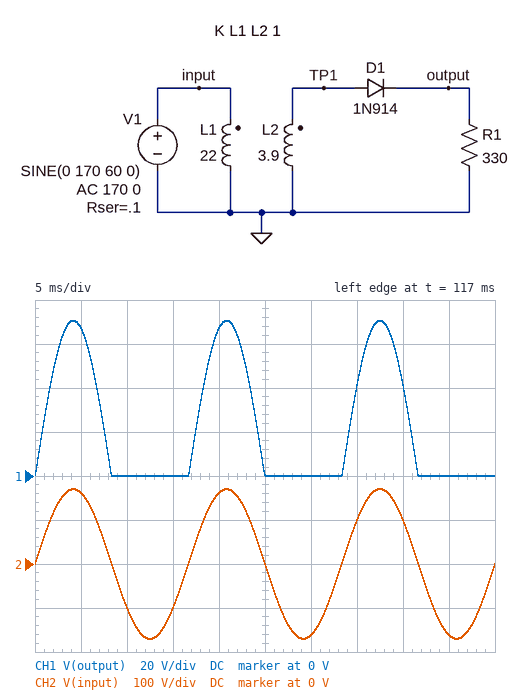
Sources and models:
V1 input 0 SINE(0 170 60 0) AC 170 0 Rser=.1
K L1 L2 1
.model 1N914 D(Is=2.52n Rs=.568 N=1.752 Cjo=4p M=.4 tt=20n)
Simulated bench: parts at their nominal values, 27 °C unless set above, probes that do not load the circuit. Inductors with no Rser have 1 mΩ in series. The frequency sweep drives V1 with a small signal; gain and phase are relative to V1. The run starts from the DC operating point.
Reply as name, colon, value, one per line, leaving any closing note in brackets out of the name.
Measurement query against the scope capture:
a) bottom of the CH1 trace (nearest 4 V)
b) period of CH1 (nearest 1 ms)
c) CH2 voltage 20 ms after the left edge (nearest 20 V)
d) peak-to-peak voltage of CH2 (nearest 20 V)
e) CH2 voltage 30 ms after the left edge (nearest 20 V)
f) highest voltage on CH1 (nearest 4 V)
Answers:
bottom of the CH1 trace: 0 V
period of CH1: 17 ms
CH2 voltage 20 ms after the left edge: 160 V
peak-to-peak voltage of CH2: 340 V
CH2 voltage 30 ms after the left edge: -160 V
highest voltage on CH1: 72 V
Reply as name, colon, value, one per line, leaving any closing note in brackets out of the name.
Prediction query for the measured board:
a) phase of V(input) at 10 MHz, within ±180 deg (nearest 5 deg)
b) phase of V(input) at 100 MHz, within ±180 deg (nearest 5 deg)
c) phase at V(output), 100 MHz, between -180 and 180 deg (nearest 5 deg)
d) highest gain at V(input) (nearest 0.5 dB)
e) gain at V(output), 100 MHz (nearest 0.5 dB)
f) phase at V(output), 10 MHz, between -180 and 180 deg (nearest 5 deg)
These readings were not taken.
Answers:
phase of V(input) at 10 MHz, within ±180 deg: 0 deg
phase of V(input) at 100 MHz, within ±180 deg: 0 deg
phase at V(output), 100 MHz, between -180 and 180 deg: 50 deg
highest gain at V(input): 0 dB
gain at V(output), 100 MHz: -11.5 dB
phase at V(output), 10 MHz, between -180 and 180 deg: 85 deg
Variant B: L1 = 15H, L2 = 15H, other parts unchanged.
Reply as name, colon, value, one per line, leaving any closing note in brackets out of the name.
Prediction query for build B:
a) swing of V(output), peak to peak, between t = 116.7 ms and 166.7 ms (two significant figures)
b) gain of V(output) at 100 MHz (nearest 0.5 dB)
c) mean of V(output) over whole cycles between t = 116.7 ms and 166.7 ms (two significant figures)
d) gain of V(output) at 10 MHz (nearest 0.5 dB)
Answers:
swing of V(output), peak to peak, between t = 116.7 ms and 166.7 ms: 170 V
gain of V(output) at 100 MHz: -4.0 dB
mean of V(output) over whole cycles between t = 116.7 ms and 166.7 ms: 54 V
gain of V(output) at 10 MHz: -21.5 dB
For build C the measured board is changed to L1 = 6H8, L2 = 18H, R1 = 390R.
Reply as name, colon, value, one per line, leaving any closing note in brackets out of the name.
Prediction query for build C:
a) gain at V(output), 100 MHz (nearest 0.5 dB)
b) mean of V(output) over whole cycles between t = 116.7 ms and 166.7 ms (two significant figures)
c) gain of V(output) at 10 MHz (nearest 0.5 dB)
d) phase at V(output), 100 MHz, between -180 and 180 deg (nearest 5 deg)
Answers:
gain at V(output), 100 MHz: 1.0 dB
mean of V(output) over whole cycles between t = 116.7 ms and 166.7 ms: 87 V
gain of V(output) at 10 MHz: -16.0 dB
phase at V(output), 100 MHz, between -180 and 180 deg: 45 deg
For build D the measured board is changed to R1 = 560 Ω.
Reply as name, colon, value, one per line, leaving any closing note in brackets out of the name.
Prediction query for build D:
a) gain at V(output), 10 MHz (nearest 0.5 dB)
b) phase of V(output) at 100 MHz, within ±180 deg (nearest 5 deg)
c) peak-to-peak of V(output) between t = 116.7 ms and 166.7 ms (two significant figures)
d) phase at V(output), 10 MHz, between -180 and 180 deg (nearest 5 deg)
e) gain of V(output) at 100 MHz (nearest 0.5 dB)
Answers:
gain at V(output), 10 MHz: -24.5 dB
phase of V(output) at 100 MHz, within ±180 deg: 35 deg
peak-to-peak of V(output) between t = 116.7 ms and 166.7 ms: 71 V
phase at V(output), 10 MHz, between -180 and 180 deg: 80 deg
gain of V(output) at 100 MHz: -9.5 dB
